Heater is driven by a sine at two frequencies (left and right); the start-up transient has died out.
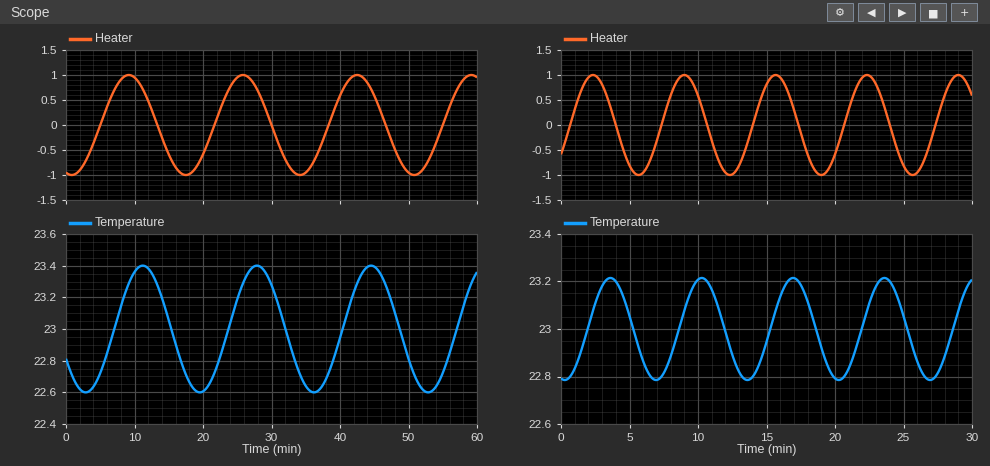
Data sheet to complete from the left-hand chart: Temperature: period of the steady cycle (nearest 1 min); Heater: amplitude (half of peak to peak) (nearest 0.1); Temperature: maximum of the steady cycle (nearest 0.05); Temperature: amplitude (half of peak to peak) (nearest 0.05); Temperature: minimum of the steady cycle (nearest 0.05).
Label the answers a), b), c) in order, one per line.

a) 17 min
b) 1.0
c) 23.40
d) 0.40
e) 22.60
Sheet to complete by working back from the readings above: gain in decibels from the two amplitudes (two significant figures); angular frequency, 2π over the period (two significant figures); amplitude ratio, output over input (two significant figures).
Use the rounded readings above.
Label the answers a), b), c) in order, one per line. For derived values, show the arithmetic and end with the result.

a) 20 log10(0.4 / 1) = -8.0 dB
b) 2π / 17 = 0.37 rad/min
c) 0.4 / 1 = 0.40
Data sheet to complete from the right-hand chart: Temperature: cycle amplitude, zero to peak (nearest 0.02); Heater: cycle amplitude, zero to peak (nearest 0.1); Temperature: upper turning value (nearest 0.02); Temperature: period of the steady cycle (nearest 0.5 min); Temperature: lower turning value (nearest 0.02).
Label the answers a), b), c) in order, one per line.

a) 0.22
b) 1.0
c) 23.22
d) 6.5 min
e) 22.78
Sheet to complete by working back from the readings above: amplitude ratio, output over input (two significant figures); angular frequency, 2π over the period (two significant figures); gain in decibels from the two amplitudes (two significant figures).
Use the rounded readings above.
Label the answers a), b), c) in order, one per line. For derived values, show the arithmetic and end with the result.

a) 0.22 / 1 = 0.22
b) 2π / 6.5 = 0.97 rad/min
c) 20 log10(0.22 / 1) = -13 dB
